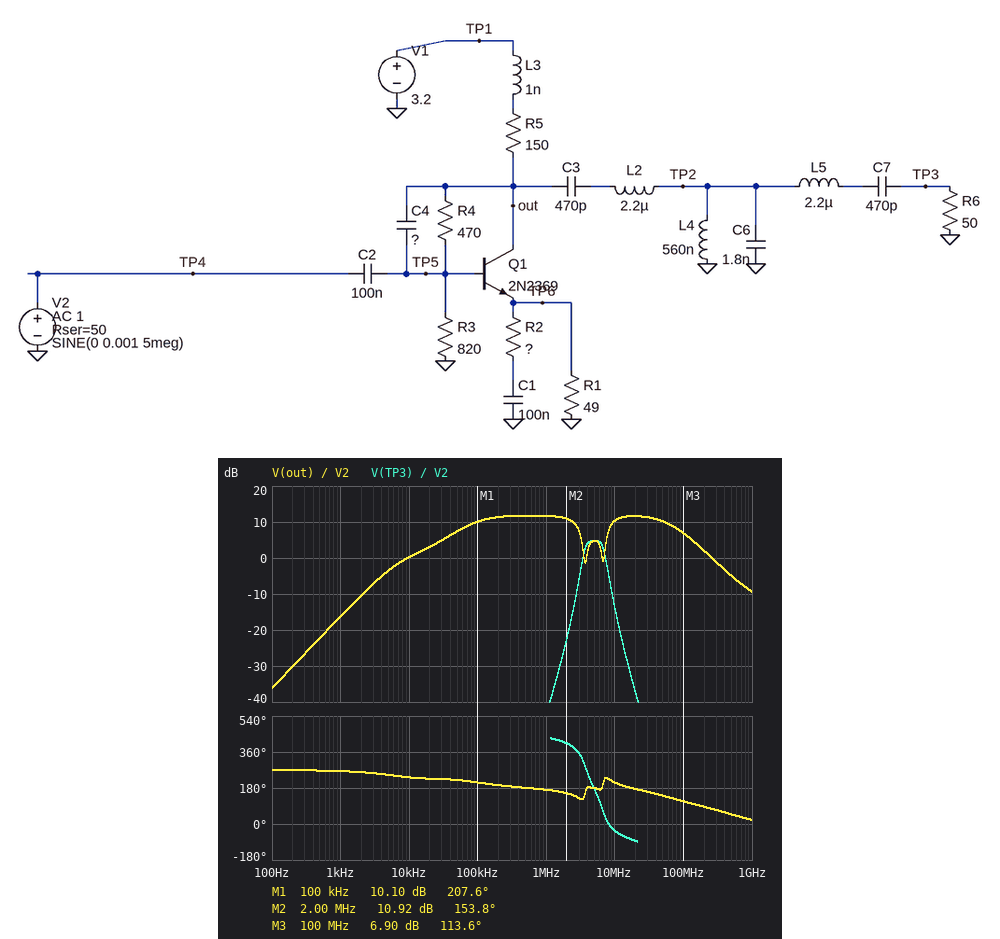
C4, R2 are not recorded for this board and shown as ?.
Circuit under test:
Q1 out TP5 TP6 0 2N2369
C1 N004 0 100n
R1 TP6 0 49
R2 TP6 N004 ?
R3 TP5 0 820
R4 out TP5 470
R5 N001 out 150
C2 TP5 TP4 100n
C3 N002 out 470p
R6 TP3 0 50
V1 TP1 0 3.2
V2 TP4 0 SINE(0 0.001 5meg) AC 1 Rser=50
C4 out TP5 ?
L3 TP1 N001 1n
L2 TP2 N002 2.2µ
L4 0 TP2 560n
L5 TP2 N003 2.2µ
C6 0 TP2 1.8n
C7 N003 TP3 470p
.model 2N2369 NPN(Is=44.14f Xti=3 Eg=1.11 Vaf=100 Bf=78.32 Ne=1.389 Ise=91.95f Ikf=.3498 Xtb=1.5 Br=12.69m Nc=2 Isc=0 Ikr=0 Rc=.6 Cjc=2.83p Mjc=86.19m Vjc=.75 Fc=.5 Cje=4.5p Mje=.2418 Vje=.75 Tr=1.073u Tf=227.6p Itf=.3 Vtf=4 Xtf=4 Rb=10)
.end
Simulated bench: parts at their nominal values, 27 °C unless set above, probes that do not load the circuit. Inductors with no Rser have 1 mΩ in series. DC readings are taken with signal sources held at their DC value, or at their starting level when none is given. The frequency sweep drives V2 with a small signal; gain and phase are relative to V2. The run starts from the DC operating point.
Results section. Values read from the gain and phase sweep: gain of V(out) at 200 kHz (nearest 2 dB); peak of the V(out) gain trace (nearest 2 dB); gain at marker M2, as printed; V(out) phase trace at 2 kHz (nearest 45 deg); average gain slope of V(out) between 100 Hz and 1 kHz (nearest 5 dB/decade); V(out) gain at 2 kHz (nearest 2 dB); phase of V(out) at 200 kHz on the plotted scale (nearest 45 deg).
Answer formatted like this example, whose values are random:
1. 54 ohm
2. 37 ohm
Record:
1. 12 dB
2. 12 dB
3. 10.92 dB
4. 270 deg
5. 20 dB/decade
6. -10 dB
7. 180 deg
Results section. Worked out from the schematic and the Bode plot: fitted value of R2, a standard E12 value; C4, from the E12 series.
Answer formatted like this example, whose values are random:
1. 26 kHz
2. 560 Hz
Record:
1. 12 Ω
2. 3.9 pF
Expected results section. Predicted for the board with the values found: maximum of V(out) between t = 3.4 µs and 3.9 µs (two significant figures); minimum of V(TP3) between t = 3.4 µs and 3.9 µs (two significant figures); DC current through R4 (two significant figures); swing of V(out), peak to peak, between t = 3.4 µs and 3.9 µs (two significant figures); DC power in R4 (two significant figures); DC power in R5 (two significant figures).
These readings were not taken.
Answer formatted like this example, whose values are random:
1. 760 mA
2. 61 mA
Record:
1. 1.8 V
2. -1.7 mV
3. 1.4 mA
4. 3.4 mV
5. 970 µW
6. 14 mW
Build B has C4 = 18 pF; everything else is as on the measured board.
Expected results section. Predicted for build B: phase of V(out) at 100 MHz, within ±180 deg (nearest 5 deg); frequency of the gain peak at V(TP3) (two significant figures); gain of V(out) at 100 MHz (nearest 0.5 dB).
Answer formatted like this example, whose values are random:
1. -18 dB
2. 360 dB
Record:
1. 85 deg
2. 5.1 MHz
3. 0 dB
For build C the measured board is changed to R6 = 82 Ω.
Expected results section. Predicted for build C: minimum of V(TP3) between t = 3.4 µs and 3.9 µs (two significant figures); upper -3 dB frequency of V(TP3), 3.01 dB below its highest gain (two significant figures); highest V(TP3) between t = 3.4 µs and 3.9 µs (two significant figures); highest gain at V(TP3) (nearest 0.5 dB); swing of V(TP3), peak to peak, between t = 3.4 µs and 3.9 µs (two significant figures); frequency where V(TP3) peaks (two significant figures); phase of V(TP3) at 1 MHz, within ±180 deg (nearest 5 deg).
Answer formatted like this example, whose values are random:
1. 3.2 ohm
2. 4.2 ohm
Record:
1. -2.2 mV
2. 6.7 MHz
3. 2.2 mV
4. 7.0 dB
5. 4.4 mV
6. 5.0 MHz
7. 65 deg
